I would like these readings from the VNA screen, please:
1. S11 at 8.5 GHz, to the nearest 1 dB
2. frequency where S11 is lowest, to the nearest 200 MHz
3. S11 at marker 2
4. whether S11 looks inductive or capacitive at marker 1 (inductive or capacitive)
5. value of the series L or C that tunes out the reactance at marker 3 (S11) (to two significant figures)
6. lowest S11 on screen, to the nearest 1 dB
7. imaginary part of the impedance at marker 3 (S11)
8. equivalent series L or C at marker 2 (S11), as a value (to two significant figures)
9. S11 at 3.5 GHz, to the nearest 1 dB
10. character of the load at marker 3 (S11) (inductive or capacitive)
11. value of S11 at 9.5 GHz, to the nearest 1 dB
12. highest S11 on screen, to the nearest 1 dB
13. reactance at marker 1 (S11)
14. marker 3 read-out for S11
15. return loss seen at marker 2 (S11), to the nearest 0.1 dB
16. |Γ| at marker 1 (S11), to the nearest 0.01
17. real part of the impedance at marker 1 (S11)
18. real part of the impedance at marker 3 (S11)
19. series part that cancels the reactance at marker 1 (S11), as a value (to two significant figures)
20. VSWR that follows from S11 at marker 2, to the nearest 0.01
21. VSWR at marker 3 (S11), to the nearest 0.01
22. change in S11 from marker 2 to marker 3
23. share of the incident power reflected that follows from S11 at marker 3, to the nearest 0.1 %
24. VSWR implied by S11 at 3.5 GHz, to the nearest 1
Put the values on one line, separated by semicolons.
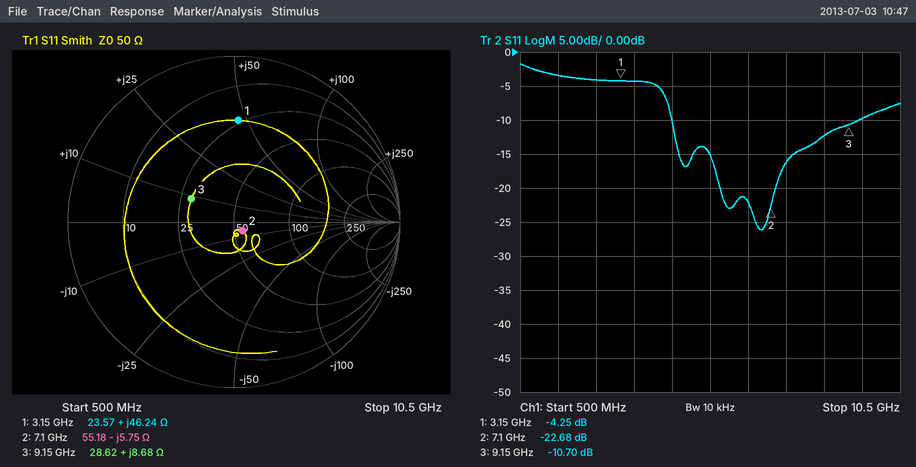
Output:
-12 dB; 6.8 GHz; -22.68 dB; inductive; 2.0 pF; -26 dB; +8.68 Ω; 3.9 pF; -4 dB; inductive; -10 dB; -2 dB; +46.24 Ω; -10.70 dB; 22.7 dB; 0.61; 23.57 Ω; 28.62 Ω; 1.1 pF; 1.16; 1.82; 11.98 dB; 8.5 %; 4
